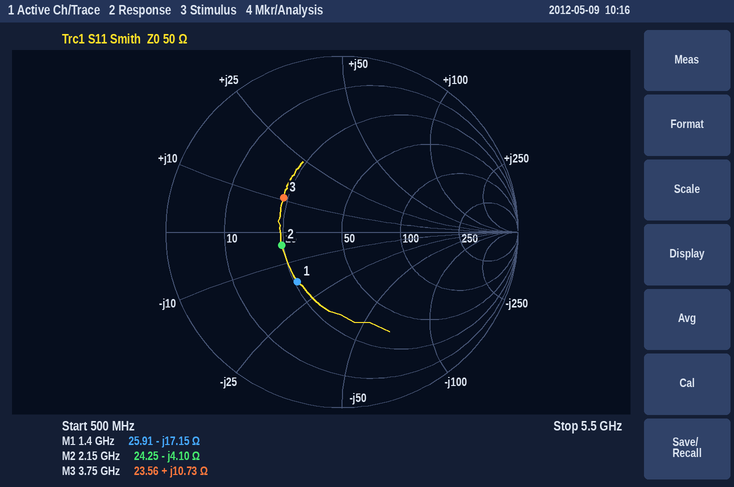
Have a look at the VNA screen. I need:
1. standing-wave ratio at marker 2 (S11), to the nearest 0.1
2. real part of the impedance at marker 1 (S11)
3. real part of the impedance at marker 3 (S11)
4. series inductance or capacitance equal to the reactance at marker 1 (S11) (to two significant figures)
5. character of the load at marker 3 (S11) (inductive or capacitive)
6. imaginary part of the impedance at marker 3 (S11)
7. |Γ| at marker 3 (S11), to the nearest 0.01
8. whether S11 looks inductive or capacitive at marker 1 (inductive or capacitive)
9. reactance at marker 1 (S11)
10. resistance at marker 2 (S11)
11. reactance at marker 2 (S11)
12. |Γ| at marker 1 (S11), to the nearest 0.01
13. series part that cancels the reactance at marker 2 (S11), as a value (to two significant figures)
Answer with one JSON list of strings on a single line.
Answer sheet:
["2.1", "25.91 Ω", "23.56 Ω", "6.6 pF", "inductive", "+10.73 Ω", "0.38", "capacitive", "-17.15 Ω", "24.25 Ω", "-4.10 Ω", "0.38", "300 pH"]
